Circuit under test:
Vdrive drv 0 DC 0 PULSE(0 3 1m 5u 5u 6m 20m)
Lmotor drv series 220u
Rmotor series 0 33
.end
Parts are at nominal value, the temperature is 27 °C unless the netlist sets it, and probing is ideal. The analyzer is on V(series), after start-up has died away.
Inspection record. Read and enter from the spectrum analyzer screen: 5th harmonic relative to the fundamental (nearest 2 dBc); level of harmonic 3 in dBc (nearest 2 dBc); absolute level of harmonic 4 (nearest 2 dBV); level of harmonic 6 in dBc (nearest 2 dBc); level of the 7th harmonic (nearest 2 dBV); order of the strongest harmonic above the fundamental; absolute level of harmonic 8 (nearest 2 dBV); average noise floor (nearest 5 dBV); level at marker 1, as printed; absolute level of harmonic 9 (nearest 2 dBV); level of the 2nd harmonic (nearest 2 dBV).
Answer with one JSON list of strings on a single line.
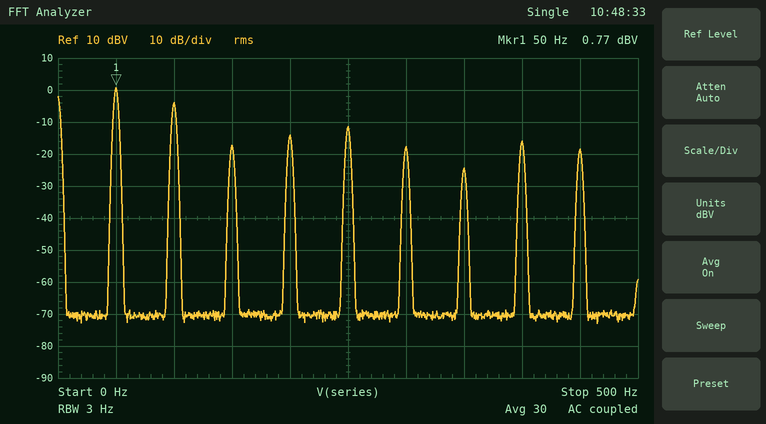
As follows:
["-12 dBc", "-18 dBc", "-14 dBV", "-18 dBc", "-24 dBV", "2", "-16 dBV", "-70 dBV", "0.77 dBV", "-18 dBV", "-4 dBV"]
